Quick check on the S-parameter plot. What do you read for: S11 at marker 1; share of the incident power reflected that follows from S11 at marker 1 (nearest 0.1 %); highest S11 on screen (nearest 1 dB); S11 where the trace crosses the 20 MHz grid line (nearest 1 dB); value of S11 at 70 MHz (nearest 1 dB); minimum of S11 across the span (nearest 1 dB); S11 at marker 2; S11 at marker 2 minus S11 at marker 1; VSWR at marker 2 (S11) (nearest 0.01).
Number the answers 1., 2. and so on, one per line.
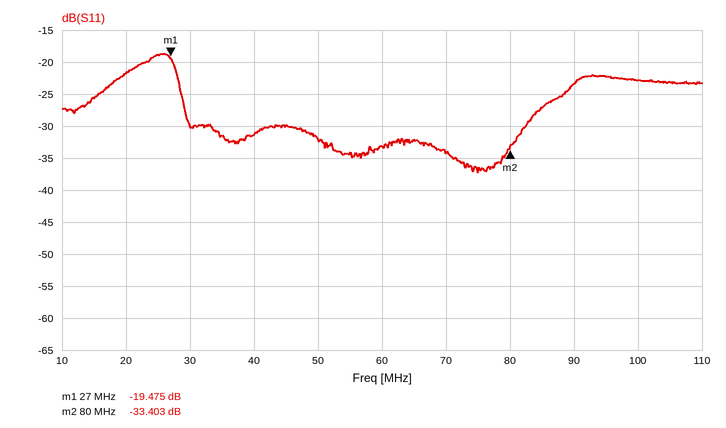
1. -19.475 dB
2. 1.1 %
3. -19 dB
4. -22 dB
5. -34 dB
6. -37 dB
7. -33.403 dB
8. -13.928 dB
9. 1.04
